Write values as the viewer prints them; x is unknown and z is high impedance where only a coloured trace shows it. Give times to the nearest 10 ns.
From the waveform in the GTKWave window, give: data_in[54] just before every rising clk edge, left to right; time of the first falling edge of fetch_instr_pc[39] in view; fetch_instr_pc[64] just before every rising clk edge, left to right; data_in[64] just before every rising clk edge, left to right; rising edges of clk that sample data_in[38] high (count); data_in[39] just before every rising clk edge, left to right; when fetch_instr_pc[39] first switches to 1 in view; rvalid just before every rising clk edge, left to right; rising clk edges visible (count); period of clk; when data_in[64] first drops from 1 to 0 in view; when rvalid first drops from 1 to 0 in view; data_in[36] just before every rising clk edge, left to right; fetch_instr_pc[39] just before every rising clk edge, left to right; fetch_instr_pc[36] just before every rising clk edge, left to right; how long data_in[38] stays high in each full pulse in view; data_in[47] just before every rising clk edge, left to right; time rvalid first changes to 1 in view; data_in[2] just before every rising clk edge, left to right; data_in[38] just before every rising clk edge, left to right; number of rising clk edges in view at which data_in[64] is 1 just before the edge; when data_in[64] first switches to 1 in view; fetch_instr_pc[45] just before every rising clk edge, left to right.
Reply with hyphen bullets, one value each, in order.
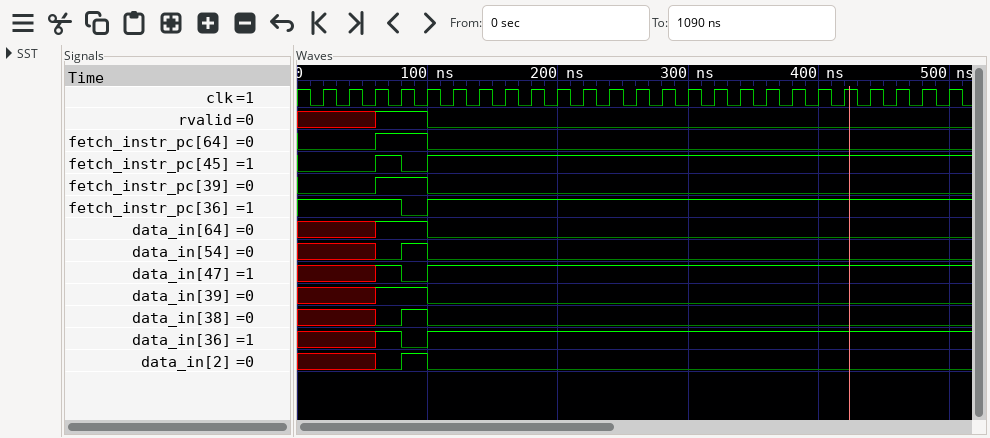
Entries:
- x x x 0 1 0 0 0 0 0 0 0 0 0 0 0 0 0 0 0 0 0 0 0 0
- 100 ns
- 0 0 0 1 1 0 0 0 0 0 0 0 0 0 0 0 0 0 0 0 0 0 0 0 0
- x x x 1 1 0 0 0 0 0 0 0 0 0 0 0 0 0 0 0 0 0 0 0 0
- 1
- x x x 1 1 0 0 0 0 0 0 0 0 0 0 0 0 0 0 0 0 0 0 0 0
- 60 ns
- x x x 1 1 0 0 0 0 0 0 0 0 0 0 0 0 0 0 0 0 0 0 0 0
- 25
- 20 ns
- 100 ns
- 100 ns
- x x x 1 0 1 1 1 1 1 1 1 1 1 1 1 1 1 1 1 1 1 1 1 1
- 0 0 0 1 1 0 0 0 0 0 0 0 0 0 0 0 0 0 0 0 0 0 0 0 0
- 1 1 1 1 0 1 1 1 1 1 1 1 1 1 1 1 1 1 1 1 1 1 1 1 1
- 20 ns
- x x x 1 0 1 1 1 1 1 1 1 1 1 1 1 1 1 1 1 1 1 1 1 1
- 60 ns
- x x x 0 1 0 0 0 0 0 0 0 0 0 0 0 0 0 0 0 0 0 0 0 0
- x x x 0 1 0 0 0 0 0 0 0 0 0 0 0 0 0 0 0 0 0 0 0 0
- 2
- 60 ns
- 0 0 0 1 0 1 1 1 1 1 1 1 1 1 1 1 1 1 1 1 1 1 1 1 1
